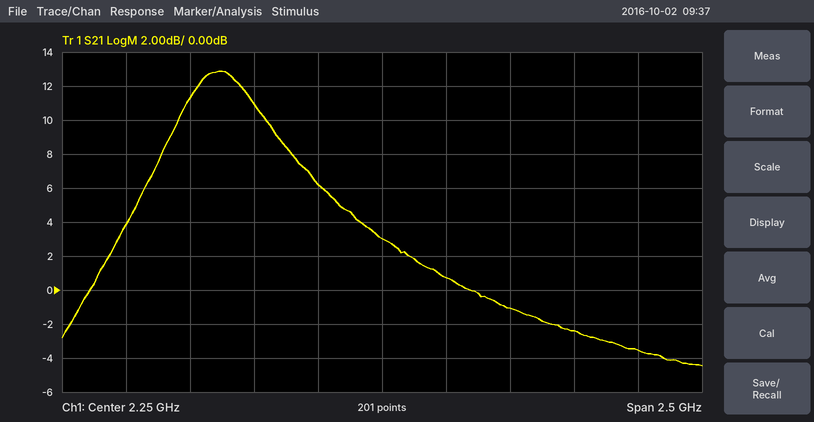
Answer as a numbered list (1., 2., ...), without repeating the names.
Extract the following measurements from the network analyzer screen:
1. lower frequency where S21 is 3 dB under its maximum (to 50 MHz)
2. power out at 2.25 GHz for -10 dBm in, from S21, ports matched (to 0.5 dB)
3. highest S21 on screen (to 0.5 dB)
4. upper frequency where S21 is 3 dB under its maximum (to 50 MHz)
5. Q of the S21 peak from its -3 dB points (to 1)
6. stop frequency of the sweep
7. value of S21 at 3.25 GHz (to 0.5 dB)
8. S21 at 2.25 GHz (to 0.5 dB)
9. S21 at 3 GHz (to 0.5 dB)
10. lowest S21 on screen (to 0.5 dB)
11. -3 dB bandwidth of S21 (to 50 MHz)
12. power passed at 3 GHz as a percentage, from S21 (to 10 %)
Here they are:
1. 1.45 GHz
2. -7.0 dBm
3. 13.0 dB
4. 1.80 GHz
5. 5
6. 3.5 GHz
7. -3.5 dB
8. 3.0 dB
9. -2.5 dB
10. -4.5 dB
11. 350 MHz
12. 60 %
